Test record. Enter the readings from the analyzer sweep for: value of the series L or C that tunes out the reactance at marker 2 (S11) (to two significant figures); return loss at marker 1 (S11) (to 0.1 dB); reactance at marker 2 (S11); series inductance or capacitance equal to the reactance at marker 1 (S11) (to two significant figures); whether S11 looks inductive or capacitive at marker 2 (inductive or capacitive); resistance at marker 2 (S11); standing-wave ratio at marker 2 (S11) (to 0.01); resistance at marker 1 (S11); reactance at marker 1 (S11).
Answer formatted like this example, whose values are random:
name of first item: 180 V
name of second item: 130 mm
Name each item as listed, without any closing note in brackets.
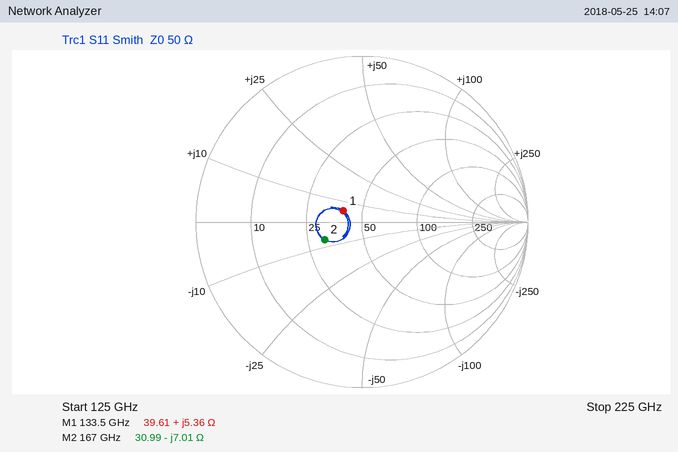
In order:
value of the series L or C that tunes out the reactance at marker 2 (S11): 6.7 pH
return loss at marker 1 (S11): 17.7 dB
reactance at marker 2: -7.01 Ω
series inductance or capacitance equal to the reactance at marker 1 (S11): 6.4 pH
whether S11 looks inductive or capacitive at marker 2: capacitive
resistance at marker 2: 30.99 Ω
standing-wave ratio at marker 2 (S11): 1.66
resistance at marker 1: 39.61 Ω
reactance at marker 1: +5.36 Ω
